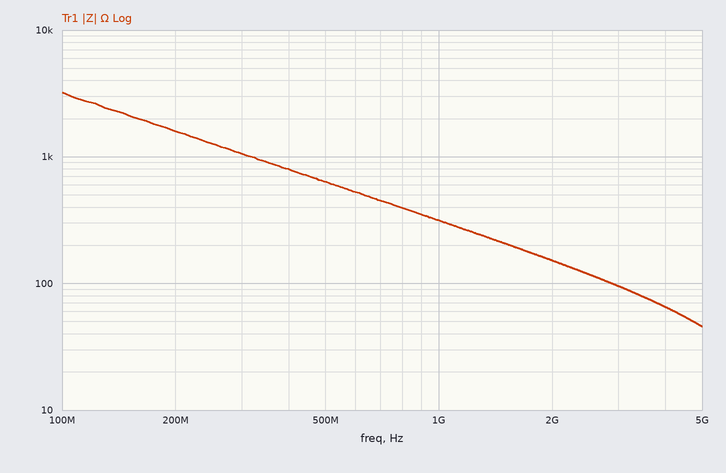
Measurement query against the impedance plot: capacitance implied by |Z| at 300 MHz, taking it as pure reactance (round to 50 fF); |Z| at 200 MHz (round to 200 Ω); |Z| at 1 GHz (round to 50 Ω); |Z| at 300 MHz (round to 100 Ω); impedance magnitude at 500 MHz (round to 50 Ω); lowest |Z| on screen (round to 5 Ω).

500 fF
1.6 kΩ
300 Ω
1.1 kΩ
650 Ω
45 Ω
